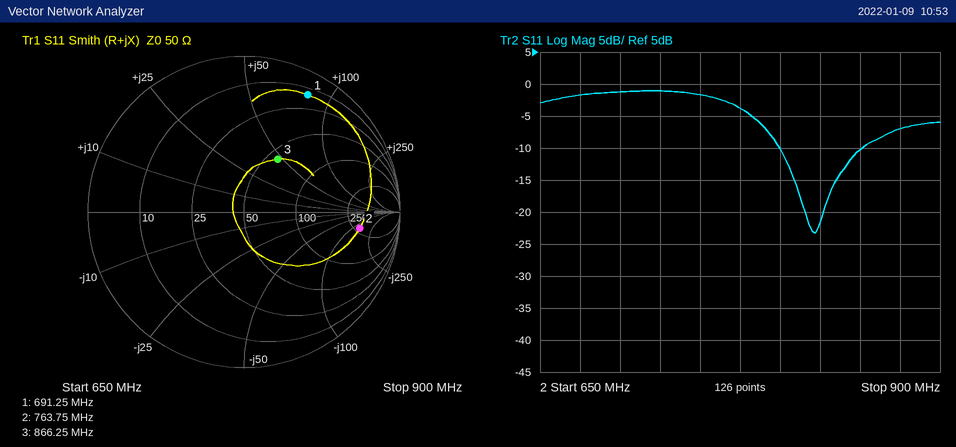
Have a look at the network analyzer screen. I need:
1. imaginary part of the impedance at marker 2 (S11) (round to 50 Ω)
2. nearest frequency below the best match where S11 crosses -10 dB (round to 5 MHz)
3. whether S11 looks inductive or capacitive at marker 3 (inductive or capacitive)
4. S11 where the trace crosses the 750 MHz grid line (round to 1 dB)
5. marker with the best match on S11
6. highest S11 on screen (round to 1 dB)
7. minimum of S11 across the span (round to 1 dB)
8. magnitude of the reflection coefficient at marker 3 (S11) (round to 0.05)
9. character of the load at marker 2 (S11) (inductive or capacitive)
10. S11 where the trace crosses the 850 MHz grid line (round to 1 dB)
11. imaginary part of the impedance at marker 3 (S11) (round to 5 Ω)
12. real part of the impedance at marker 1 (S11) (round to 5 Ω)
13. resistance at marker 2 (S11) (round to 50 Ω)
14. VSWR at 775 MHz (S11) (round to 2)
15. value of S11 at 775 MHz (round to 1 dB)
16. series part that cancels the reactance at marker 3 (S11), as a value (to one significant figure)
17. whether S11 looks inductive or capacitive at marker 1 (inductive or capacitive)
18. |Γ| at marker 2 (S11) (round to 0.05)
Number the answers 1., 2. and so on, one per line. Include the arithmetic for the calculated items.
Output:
1. -150 Ω
2. 800 MHz
3. inductive
4. -2 dB
5. marker 3
6. -1 dB
7. -23 dB
8. 0.40
9. capacitive
10. -10 dB
11. +45 Ω
12. 15 Ω
13. 300 Ω
14. |Γ| = 10^(-4/20) = 0.6310; VSWR = (1 + 0.6310)/(1 − 0.6310) ≈ 4
15. -4 dB
16. C = 1/(2π × 866.25 MHz × 45 Ω) ≈ 4 pF
17. inductive
18. 0.75
